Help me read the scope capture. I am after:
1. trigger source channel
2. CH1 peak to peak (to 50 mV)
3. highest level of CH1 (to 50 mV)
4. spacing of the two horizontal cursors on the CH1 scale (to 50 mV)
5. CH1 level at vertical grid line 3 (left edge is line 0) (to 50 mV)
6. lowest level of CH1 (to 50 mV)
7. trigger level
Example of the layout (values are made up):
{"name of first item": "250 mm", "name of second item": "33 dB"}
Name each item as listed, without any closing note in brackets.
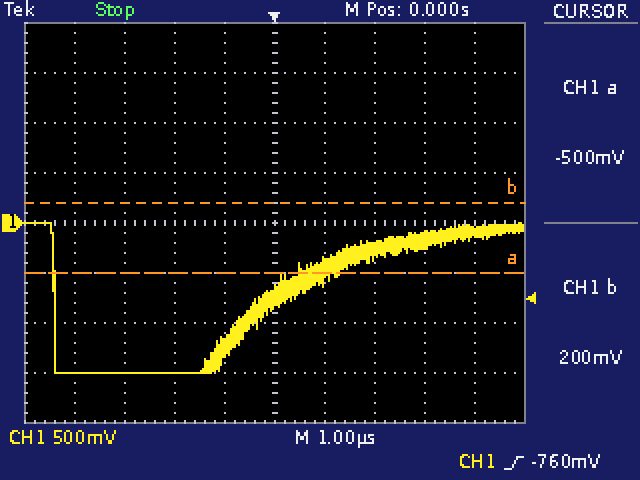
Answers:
{"trigger source channel": "CH1", "CH1 peak to peak": "1.50 V", "highest level of CH1": "0 mV", "spacing of the two horizontal cursors on the CH1 scale": "700 mV", "CH1 level at vertical grid line 3 (left edge is line 0)": "-1.50 V", "lowest level of CH1": "-1.50 V", "trigger level": "-760 mV"}
